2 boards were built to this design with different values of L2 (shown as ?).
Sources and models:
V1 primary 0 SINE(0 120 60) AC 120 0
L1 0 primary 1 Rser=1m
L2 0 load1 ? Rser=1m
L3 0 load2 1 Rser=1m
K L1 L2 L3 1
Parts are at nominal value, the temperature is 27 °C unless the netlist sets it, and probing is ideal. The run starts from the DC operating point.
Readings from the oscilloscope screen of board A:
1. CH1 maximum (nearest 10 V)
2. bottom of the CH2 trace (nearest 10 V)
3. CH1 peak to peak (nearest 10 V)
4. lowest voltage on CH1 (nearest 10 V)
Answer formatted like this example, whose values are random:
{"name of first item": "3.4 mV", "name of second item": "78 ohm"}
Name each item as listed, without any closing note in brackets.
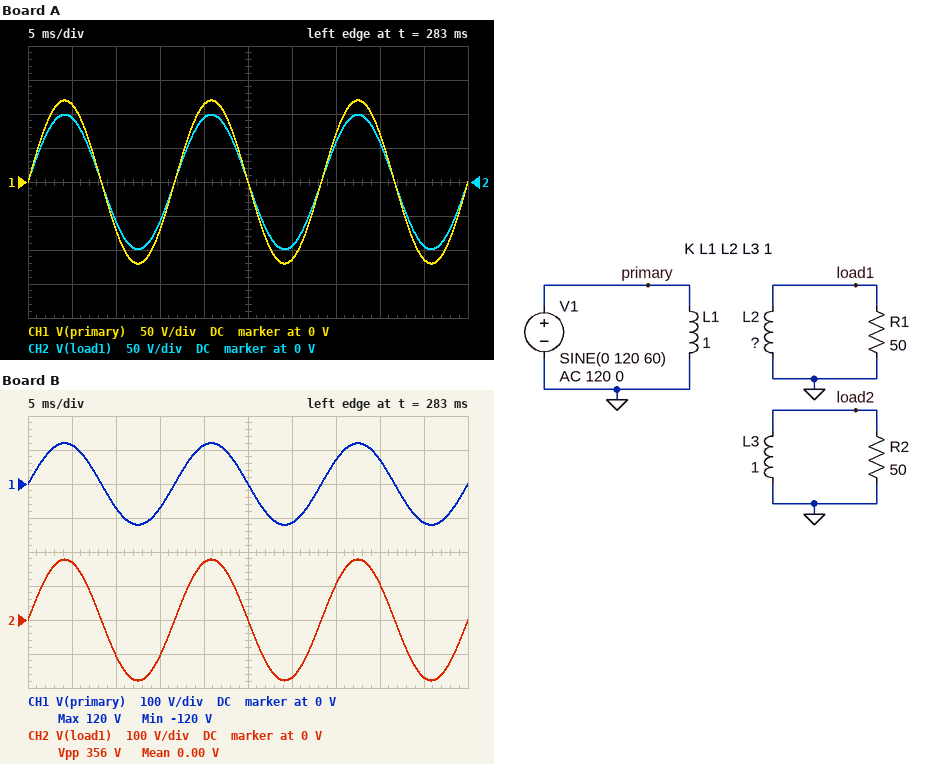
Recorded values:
{"CH1 maximum": "120 V", "bottom of the CH2 trace": "-100 V", "CH1 peak to peak": "240 V", "lowest voltage on CH1": "-120 V"}
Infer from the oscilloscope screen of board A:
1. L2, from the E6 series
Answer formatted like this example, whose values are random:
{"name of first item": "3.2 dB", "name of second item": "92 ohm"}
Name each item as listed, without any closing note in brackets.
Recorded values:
{"L2, from the E6 series": "680 mH"}
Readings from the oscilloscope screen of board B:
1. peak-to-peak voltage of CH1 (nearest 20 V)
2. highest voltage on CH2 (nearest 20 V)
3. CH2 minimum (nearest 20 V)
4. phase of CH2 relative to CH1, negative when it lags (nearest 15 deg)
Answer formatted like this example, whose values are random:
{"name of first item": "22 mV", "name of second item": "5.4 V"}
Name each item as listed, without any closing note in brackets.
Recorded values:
{"peak-to-peak voltage of CH1": "240 V", "highest voltage on CH2": "180 V", "CH2 minimum": "-180 V", "phase of CH2 relative to CH1, negative when it lags": "0 deg"}
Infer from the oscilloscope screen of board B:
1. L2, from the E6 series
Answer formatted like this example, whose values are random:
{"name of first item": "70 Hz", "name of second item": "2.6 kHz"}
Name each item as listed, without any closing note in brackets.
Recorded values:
{"L2, from the E6 series": "2.2 H"}
